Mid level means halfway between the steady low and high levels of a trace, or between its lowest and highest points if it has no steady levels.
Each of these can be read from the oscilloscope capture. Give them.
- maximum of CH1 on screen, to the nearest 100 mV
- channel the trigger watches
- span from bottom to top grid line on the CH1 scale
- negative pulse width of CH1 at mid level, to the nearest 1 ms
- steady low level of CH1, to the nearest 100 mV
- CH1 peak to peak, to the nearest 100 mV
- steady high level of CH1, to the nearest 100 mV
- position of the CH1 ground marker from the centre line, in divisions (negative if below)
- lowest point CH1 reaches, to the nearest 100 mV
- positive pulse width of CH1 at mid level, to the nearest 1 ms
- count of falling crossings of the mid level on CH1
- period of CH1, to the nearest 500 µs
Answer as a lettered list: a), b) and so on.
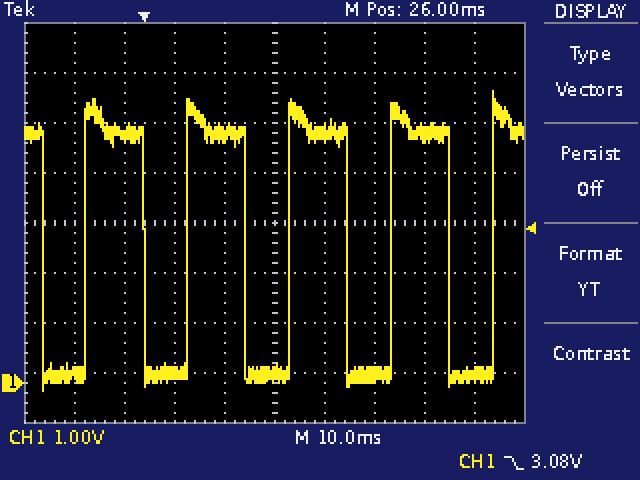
a) 5.8 V
b) CH1
c) 8 V
d) 9 ms
e) 200 mV
f) 6.0 V
g) 5.0 V
h) -3.2 div
i) -200 mV
j) 12 ms
k) 5
l) 20.5 ms
